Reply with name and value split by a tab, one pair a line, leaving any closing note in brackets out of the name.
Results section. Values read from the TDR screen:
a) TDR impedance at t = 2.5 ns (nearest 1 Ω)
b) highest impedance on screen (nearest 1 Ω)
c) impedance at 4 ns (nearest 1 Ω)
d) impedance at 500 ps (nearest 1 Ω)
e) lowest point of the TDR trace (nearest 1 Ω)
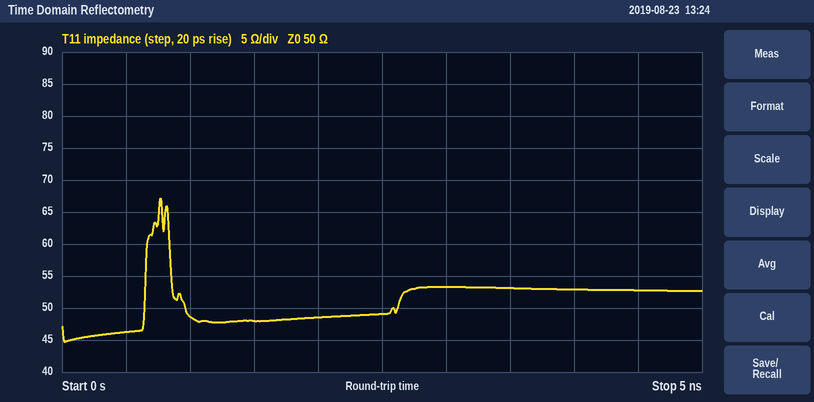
TDR impedance at t = 2.5 ns	49 Ω
highest impedance on screen	67 Ω
impedance at 4 ns	53 Ω
impedance at 500 ps	46 Ω
lowest point of the TDR trace	45 Ω
